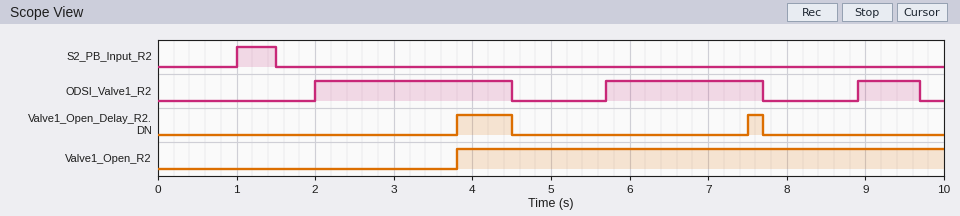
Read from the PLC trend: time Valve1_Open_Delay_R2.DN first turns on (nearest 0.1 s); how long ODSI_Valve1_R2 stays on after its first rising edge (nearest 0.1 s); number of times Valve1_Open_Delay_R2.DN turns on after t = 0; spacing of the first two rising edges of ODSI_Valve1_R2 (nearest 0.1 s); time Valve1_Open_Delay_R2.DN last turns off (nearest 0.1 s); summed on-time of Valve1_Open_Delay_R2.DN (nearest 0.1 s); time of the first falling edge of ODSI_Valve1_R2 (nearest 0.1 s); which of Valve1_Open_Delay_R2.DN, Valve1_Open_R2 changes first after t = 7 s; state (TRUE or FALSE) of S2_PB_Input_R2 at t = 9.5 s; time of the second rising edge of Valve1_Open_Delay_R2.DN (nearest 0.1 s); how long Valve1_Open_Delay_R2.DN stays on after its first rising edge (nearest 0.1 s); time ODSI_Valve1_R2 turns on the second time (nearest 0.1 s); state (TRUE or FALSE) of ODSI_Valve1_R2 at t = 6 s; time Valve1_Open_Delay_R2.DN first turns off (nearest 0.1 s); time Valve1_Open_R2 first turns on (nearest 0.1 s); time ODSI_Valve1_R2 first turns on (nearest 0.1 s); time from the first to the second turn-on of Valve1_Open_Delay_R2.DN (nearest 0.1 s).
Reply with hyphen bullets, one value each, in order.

- 3.8 s
- 2.5 s
- 2
- 3.7 s
- 7.7 s
- 0.9 s
- 4.5 s
- Valve1_Open_Delay_R2.DN
- FALSE
- 7.5 s
- 0.7 s
- 5.7 s
- TRUE
- 4.5 s
- 3.8 s
- 2.0 s
- 3.7 s
